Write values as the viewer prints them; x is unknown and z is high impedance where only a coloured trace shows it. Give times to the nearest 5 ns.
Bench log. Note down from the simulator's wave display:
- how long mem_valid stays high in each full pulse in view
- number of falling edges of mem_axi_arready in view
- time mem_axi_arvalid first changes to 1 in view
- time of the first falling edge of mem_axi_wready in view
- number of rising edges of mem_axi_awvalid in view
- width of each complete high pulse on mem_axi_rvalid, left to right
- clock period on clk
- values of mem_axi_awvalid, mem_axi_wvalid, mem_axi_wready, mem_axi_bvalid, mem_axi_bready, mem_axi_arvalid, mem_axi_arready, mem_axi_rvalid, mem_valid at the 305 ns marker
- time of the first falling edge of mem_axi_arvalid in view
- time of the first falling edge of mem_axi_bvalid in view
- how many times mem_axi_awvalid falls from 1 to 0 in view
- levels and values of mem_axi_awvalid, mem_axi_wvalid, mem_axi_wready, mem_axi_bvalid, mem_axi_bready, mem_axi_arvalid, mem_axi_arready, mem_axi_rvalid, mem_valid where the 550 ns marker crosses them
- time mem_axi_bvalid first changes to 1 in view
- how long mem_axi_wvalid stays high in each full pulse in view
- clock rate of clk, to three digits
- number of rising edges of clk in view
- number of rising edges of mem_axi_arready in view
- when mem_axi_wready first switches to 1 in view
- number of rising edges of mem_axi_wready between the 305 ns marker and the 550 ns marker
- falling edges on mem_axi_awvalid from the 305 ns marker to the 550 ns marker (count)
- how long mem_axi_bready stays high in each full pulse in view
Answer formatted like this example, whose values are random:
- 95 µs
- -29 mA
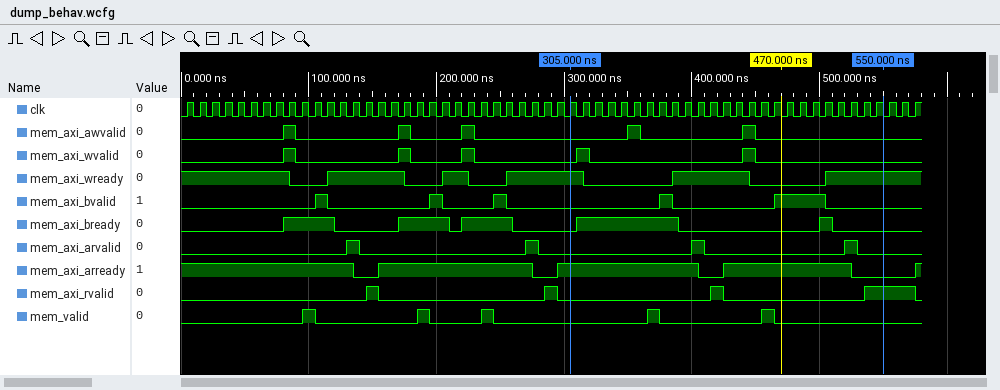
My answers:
- 10 ns, 10 ns, 10 ns, 10 ns, 10 ns
- 4
- 130 ns
- 85 ns
- 5
- 10 ns, 10 ns, 10 ns, 40 ns
- 10 ns
- mem_axi_awvalid=0, mem_axi_wvalid=0, mem_axi_wready=1, mem_axi_bvalid=0, mem_axi_bready=0, mem_axi_arvalid=0, mem_axi_arready=1, mem_axi_rvalid=0, mem_valid=0
- 140 ns
- 115 ns
- 5
- mem_axi_awvalid=0, mem_axi_wvalid=0, mem_axi_wready=1, mem_axi_bvalid=0, mem_axi_bready=0, mem_axi_arvalid=0, mem_axi_arready=0, mem_axi_rvalid=1, mem_valid=0
- 105 ns
- 10 ns, 10 ns, 10 ns, 10 ns, 10 ns
- 100 MHz
- 58
- 4
- 115 ns
- 2
- 2
- 40 ns, 40 ns, 40 ns, 80 ns, 10 ns
